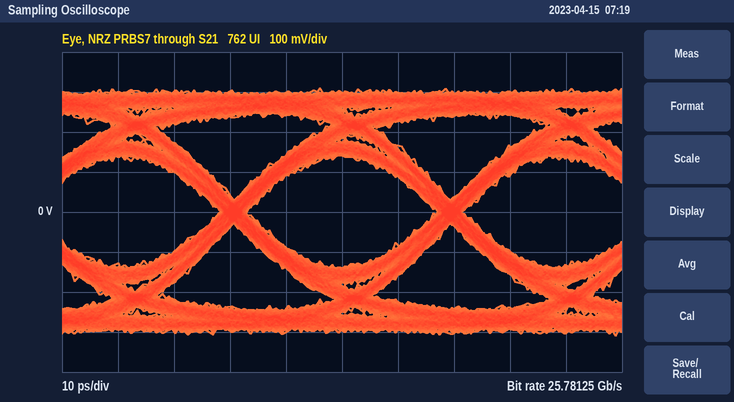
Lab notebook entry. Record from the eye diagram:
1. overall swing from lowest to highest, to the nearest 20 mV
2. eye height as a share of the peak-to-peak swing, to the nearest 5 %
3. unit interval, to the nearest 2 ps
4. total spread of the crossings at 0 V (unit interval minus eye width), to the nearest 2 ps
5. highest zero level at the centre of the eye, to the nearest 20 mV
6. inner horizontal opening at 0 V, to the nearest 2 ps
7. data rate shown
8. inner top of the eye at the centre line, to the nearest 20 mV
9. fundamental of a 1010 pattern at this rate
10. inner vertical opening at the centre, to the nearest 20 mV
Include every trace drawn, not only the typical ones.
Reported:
620 mV
45 %
38 ps
4 ps
-140 mV
34 ps
25.78125 Gb/s
140 mV
12.89062 GHz
280 mV
